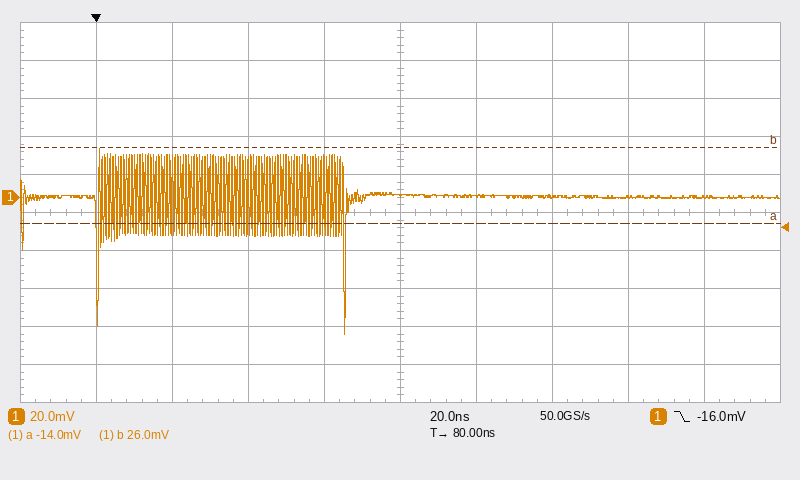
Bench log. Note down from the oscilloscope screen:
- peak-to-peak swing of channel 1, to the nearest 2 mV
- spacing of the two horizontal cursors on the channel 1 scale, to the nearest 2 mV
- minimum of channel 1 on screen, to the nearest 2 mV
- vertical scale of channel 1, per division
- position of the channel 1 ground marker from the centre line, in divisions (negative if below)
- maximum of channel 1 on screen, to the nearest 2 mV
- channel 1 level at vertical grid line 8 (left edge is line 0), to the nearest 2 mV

98 mV
40 mV
-72 mV
20 mV
+0.4 div
26 mV
0 mV
